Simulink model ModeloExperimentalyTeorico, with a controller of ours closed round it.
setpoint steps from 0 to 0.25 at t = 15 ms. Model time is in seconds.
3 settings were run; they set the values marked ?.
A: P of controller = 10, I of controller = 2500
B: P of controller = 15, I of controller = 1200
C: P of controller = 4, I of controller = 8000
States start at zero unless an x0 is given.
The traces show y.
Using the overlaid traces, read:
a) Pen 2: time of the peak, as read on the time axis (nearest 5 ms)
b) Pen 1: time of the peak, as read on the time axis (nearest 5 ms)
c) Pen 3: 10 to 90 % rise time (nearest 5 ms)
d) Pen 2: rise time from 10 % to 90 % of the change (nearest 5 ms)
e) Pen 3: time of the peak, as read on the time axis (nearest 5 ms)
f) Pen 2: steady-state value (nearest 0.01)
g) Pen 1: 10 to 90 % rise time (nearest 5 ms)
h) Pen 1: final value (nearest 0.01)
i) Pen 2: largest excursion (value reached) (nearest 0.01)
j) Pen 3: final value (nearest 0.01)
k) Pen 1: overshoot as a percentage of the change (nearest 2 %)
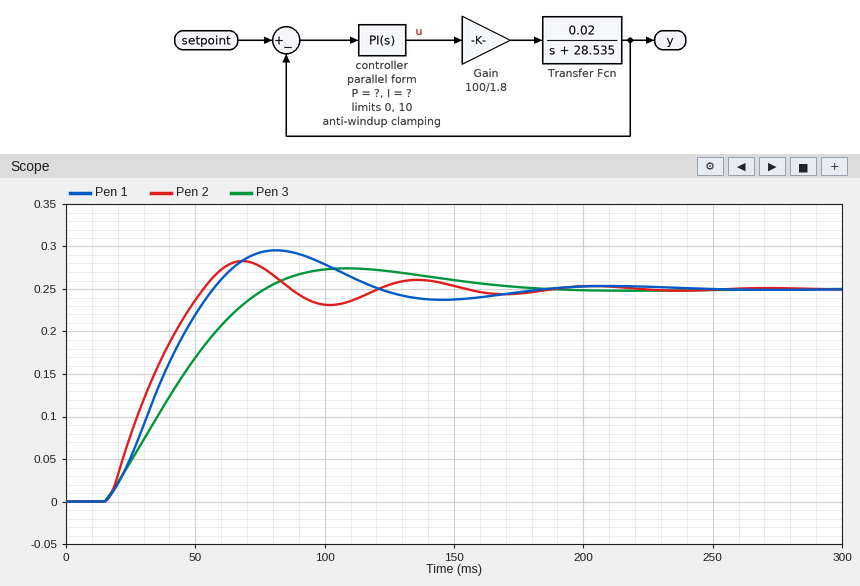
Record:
70 ms
80 ms
45 ms
30 ms
110 ms
0.25
30 ms
0.25
0.28
0.25
18 %
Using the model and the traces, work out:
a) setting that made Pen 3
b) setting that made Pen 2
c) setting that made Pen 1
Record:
B
C
A
